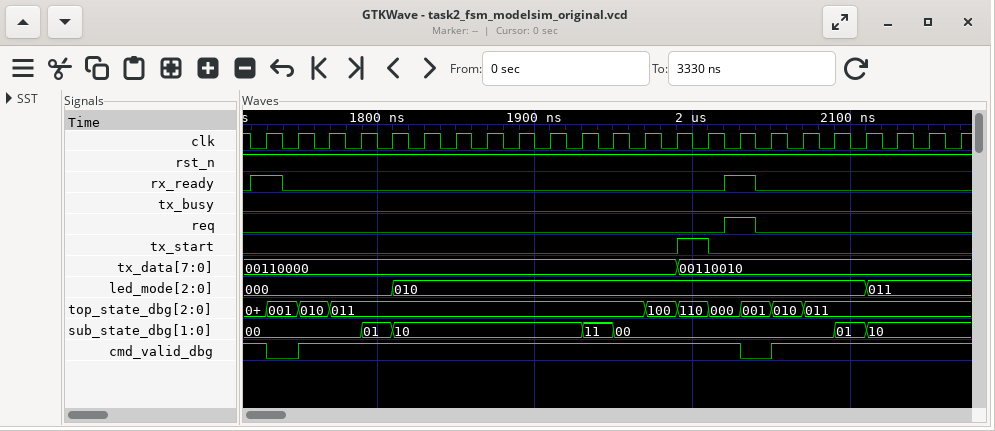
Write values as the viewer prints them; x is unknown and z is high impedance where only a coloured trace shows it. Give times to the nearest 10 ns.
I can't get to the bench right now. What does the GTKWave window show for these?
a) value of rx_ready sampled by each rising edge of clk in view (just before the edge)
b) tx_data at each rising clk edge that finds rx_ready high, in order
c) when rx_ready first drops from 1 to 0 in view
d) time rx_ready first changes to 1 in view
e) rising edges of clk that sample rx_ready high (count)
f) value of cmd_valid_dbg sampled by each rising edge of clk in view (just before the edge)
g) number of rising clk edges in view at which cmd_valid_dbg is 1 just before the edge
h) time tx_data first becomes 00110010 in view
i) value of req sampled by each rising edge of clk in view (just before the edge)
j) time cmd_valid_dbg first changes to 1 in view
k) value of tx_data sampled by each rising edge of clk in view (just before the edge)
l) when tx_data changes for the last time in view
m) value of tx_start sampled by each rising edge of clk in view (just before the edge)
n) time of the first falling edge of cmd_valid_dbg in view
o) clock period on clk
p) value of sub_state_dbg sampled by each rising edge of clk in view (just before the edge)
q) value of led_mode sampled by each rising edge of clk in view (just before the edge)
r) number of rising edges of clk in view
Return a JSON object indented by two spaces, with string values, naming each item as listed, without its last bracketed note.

{
  "value of rx_ready sampled by each rising edge of clk in view": "1 0 0 0 0 0 0 0 0 0 0 0 0 0 0 1 0 0 0 0 0 0 0",
  "tx_data at each rising clk edge that finds rx_ready high, in order": "00110000, 00110010",
  "when rx_ready first drops from 1 to 0 in view": "1740 ns",
  "time rx_ready first changes to 1 in view": "1720 ns",
  "rising edges of clk that sample rx_ready high": "2",
  "value of cmd_valid_dbg sampled by each rising edge of clk in view": "1 0 1 1 1 1 1 1 1 1 1 1 1 1 1 1 0 1 1 1 1 1 1",
  "number of rising clk edges in view at which cmd_valid_dbg is 1 just before the edge": "21",
  "time tx_data first becomes 00110010 in view": "1990 ns",
  "value of req sampled by each rising edge of clk in view": "0 0 0 0 0 0 0 0 0 0 0 0 0 0 0 1 0 0 0 0 0 0 0",
  "time cmd_valid_dbg first changes to 1 in view": "1750 ns",
  "value of tx_data sampled by each rising edge of clk in view": "00110000, 00110000, 00110000, 00110000, 00110000, 00110000, 00110000, 00110000, 00110000, 00110000, 00110000, 00110000, 00110000, 00110000, 00110010, 00110010, 00110010, 00110010, 00110010, 00110010, 00110010, 00110010, 00110010",
  "when tx_data changes for the last time in view": "1990 ns",
  "value of tx_start sampled by each rising edge of clk in view": "0 0 0 0 0 0 0 0 0 0 0 0 0 0 1 0 0 0 0 0 0 0 0",
  "time of the first falling edge of cmd_valid_dbg in view": "1730 ns",
  "clock period on clk": "20 ns",
  "value of sub_state_dbg sampled by each rising edge of clk in view": "00, 00, 00, 00, 01, 10, 10, 10, 10, 10, 10, 11, 00, 00, 00, 00, 00, 00, 00, 01, 10, 10, 10",
  "value of led_mode sampled by each rising edge of clk in view": "000, 000, 000, 000, 000, 010, 010, 010, 010, 010, 010, 010, 010, 010, 010, 010, 010, 010, 010, 010, 011, 011, 011",
  "number of rising edges of clk in view": "23"
}
